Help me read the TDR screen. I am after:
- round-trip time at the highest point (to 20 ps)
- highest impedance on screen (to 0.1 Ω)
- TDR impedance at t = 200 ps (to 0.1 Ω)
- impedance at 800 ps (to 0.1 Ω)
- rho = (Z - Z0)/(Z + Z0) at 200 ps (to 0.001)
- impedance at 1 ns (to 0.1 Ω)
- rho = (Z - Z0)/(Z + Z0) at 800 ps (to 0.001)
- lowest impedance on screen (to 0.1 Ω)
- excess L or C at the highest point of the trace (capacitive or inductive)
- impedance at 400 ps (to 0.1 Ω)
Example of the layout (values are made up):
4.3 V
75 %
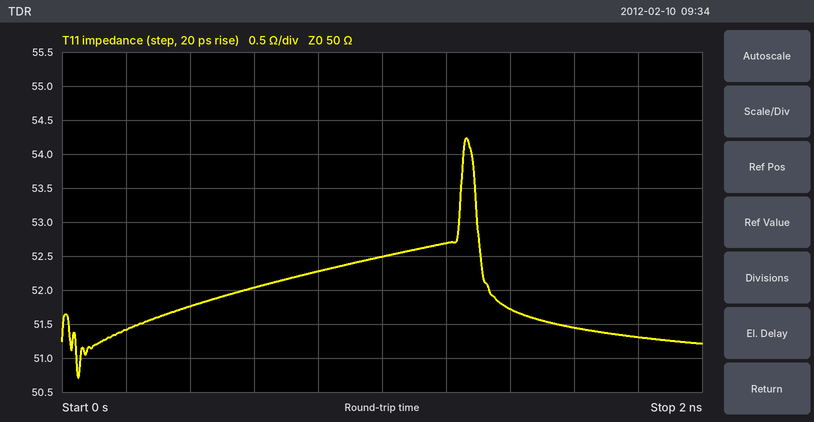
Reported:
1.26 ns
54.2 Ω
51.4 Ω
52.3 Ω
+0.014
52.5 Ω
+0.022
50.7 Ω
inductive
51.8 Ω
